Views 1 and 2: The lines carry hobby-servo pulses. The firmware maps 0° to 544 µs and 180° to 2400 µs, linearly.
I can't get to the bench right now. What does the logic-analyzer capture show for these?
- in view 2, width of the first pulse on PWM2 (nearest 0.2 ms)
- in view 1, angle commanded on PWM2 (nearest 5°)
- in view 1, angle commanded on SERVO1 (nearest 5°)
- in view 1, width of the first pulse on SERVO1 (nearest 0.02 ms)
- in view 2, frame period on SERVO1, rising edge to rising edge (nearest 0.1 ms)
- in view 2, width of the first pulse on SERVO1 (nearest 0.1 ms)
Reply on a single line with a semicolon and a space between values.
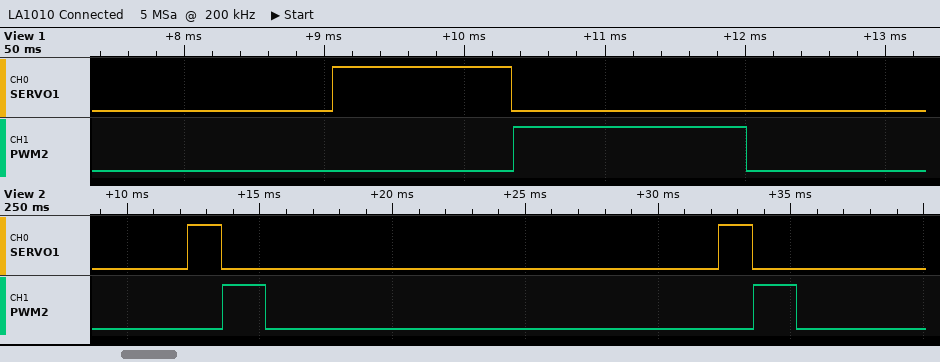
1.6 ms; 110°; 70°; 1.28 ms; 20.0 ms; 1.3 ms
